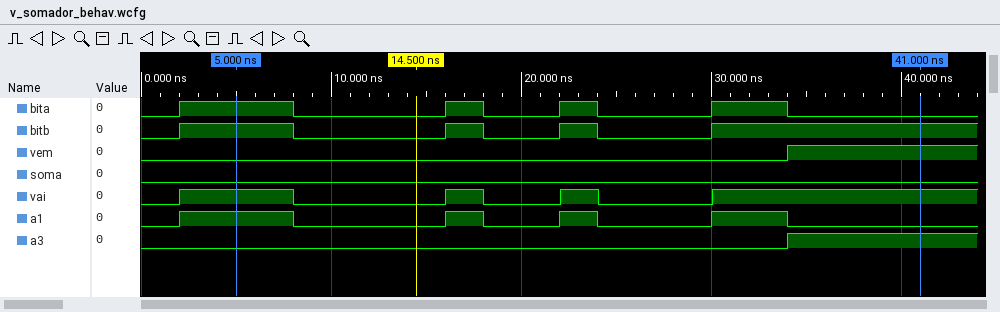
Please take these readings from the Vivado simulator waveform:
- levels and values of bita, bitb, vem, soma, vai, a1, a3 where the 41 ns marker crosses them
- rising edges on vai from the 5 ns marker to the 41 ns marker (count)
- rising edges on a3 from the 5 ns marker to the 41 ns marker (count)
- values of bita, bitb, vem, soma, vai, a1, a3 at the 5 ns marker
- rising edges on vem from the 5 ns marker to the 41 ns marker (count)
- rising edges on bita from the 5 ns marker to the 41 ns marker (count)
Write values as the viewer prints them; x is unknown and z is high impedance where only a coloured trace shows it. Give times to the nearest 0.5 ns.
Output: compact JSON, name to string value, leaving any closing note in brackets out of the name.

{"levels and values of bita, bitb, vem, soma, vai, a1, a3 where the 41 ns marker crosses them": "bita=0, bitb=1, vem=1, soma=0, vai=1, a1=0, a3=1", "rising edges on vai from the 5 ns marker to the 41 ns marker": "3", "rising edges on a3 from the 5 ns marker to the 41 ns marker": "1", "values of bita, bitb, vem, soma, vai, a1, a3 at the 5 ns marker": "bita=1, bitb=1, vem=0, soma=0, vai=1, a1=1, a3=0", "rising edges on vem from the 5 ns marker to the 41 ns marker": "1", "rising edges on bita from the 5 ns marker to the 41 ns marker": "3"}
